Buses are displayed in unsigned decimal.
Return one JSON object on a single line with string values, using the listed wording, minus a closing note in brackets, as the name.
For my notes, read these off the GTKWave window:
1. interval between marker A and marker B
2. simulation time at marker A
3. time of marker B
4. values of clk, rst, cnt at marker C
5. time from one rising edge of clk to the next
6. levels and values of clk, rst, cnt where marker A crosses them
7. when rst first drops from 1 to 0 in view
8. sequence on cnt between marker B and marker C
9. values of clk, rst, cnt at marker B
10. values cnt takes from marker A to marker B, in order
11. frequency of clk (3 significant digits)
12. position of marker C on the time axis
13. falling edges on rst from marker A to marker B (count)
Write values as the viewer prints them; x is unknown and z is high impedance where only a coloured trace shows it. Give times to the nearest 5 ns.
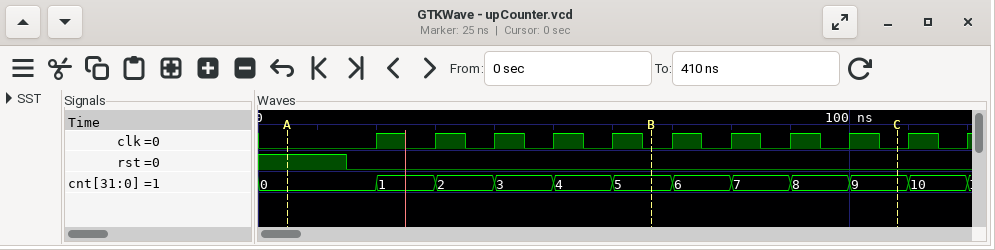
{"interval between marker A and marker B": "60 ns", "simulation time at marker A": "5 ns", "time of marker B": "65 ns", "values of clk, rst, cnt at marker C": "clk=0, rst=0, cnt=9", "time from one rising edge of clk to the next": "10 ns", "levels and values of clk, rst, cnt where marker A crosses them": "clk=0, rst=1, cnt=0", "when rst first drops from 1 to 0 in view": "15 ns", "sequence on cnt between marker B and marker C": "5, 6, 7, 8, 9", "values of clk, rst, cnt at marker B": "clk=0, rst=0, cnt=5", "values cnt takes from marker A to marker B, in order": "0, 1, 2, 3, 4, 5", "frequency of clk": "100 MHz", "position of marker C on the time axis": "110 ns", "falling edges on rst from marker A to marker B": "1"}
